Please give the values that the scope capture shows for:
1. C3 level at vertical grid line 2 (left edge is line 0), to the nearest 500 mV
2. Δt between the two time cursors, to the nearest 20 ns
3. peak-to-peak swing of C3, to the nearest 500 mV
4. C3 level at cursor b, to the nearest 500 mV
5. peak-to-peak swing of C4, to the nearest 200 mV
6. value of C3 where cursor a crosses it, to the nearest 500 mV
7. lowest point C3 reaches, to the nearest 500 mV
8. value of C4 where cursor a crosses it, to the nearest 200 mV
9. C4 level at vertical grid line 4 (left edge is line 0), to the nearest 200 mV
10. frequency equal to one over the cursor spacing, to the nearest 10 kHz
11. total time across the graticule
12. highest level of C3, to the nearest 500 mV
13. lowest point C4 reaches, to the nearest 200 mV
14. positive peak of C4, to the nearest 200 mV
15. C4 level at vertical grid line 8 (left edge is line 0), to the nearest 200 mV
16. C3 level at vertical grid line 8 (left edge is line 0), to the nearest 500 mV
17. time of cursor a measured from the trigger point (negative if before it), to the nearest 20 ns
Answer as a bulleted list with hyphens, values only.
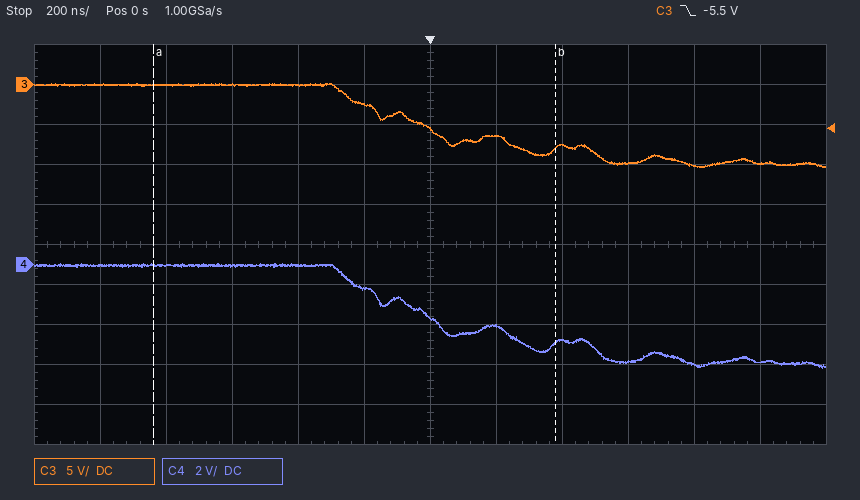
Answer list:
- 0.0 V
- 1.22 µs
- 10.5 V
- -8.0 V
- 5.2 V
- 0.0 V
- -10.5 V
- 0.0 V
- 0.0 V
- 820 kHz
- 2.4 µs
- 0.0 V
- -5.2 V
- 0.0 V
- -3.8 V
- -7.5 V
- -840 ns
